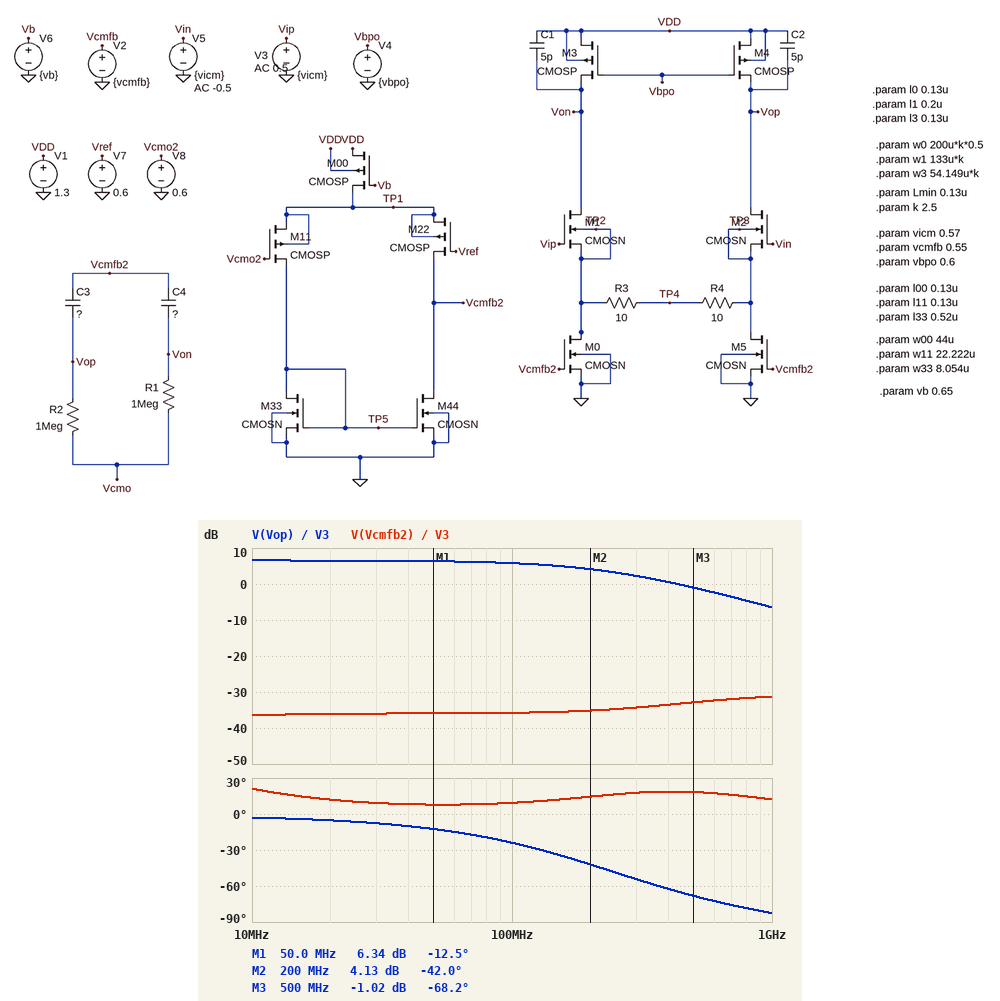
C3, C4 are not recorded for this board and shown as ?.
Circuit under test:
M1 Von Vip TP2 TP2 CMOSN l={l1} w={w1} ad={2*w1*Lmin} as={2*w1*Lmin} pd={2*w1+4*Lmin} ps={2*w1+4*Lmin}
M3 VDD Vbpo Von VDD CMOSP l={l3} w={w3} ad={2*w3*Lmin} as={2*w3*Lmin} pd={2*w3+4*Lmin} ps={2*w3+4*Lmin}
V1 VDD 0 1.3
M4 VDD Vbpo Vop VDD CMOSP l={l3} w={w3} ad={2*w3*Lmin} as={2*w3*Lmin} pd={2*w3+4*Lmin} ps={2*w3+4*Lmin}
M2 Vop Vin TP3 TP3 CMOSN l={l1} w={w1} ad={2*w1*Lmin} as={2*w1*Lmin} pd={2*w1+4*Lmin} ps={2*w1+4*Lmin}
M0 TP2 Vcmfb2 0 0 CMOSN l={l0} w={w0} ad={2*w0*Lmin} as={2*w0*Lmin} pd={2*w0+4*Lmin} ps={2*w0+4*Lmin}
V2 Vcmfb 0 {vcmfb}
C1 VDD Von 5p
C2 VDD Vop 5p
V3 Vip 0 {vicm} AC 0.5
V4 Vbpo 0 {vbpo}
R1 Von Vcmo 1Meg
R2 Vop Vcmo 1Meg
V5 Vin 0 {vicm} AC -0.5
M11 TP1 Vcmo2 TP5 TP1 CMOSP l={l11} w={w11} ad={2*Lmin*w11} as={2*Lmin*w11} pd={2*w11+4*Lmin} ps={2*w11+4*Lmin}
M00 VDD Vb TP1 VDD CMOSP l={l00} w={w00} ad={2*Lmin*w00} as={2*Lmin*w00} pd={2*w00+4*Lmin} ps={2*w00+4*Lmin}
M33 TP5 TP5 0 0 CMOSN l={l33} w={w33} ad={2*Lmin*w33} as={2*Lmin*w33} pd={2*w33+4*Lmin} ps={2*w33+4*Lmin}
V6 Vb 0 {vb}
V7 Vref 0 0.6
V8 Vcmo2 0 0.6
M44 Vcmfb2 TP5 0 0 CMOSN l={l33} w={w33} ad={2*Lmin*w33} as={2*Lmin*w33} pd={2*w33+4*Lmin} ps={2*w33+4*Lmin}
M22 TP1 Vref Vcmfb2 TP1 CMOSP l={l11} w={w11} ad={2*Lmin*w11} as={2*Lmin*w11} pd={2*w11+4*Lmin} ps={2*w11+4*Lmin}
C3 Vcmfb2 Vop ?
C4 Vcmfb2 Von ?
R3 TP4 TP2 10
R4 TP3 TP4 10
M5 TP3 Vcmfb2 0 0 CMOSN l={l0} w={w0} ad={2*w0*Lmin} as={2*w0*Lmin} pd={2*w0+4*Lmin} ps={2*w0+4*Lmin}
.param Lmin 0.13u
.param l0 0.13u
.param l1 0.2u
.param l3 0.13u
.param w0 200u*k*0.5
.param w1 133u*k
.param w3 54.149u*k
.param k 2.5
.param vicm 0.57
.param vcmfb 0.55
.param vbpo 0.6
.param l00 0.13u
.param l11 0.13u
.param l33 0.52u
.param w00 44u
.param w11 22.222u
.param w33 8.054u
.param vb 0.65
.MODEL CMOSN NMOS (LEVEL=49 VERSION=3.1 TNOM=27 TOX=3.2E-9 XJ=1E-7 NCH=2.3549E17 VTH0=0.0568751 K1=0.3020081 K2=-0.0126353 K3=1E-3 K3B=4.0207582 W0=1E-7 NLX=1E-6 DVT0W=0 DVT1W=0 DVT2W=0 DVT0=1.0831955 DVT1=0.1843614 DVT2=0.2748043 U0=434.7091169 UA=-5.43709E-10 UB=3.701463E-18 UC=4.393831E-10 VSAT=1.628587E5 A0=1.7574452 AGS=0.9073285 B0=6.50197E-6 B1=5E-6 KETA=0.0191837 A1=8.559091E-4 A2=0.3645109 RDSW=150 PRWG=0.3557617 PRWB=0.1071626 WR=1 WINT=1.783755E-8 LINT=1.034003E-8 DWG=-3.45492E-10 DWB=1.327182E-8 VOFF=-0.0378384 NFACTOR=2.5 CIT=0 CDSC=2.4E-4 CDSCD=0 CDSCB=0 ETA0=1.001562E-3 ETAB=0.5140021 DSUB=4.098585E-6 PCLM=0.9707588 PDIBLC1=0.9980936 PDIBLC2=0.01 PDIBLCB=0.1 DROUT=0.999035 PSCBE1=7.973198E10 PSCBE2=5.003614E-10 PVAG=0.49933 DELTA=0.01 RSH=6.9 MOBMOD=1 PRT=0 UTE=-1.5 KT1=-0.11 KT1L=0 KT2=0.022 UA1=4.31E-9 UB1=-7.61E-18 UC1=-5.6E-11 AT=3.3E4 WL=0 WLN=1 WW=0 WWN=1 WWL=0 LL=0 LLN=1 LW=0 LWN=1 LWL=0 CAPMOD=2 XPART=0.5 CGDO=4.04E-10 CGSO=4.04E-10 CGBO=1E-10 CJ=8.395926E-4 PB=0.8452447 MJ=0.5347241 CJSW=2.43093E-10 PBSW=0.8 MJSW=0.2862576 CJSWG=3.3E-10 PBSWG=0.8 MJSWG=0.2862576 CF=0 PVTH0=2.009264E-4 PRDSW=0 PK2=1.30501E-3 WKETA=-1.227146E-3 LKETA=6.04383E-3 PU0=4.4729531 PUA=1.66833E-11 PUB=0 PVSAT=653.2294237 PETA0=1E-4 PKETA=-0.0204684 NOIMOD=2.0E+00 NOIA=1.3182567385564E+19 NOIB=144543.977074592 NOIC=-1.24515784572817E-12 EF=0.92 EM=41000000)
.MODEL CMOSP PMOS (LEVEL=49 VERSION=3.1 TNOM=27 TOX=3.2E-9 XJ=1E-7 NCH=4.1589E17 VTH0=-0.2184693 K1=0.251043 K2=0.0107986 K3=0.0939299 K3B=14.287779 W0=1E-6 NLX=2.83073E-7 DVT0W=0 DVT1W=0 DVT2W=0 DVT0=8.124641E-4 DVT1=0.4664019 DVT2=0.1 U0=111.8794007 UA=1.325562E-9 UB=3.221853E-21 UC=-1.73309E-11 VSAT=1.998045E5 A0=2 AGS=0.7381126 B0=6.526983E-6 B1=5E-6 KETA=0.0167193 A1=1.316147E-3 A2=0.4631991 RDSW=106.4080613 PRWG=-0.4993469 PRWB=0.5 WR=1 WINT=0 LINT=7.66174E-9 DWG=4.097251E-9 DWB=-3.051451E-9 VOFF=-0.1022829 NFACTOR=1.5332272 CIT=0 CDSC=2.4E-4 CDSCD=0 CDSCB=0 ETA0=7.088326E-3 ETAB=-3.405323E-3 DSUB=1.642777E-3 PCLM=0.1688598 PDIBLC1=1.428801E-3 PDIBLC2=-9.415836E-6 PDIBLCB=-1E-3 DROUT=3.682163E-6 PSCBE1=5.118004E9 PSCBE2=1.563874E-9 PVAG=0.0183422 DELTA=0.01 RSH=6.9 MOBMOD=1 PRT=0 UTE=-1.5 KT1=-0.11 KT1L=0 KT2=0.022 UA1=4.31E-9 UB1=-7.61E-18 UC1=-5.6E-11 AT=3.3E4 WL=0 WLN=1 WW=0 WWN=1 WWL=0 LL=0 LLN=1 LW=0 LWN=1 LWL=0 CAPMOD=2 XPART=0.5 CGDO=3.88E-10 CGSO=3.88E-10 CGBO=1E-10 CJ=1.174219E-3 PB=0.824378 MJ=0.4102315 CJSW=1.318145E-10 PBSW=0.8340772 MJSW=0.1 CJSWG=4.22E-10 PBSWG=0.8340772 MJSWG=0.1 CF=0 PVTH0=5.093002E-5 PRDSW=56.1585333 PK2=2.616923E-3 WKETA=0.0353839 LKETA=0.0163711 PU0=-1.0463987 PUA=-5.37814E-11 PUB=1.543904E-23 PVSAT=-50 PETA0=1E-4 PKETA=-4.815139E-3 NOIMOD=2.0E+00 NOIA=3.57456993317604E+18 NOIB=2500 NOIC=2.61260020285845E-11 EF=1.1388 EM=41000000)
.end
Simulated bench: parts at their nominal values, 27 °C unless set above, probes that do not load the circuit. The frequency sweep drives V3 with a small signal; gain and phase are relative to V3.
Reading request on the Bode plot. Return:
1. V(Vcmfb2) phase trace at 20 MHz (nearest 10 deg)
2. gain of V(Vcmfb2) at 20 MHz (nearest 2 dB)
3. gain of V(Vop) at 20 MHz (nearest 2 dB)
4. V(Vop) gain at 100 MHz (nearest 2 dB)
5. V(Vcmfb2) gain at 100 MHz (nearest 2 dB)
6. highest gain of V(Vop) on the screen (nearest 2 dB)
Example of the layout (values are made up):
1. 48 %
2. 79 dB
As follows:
1. 10 deg
2. -36 dB
3. 6 dB
4. 6 dB
5. -36 dB
6. 6 dB
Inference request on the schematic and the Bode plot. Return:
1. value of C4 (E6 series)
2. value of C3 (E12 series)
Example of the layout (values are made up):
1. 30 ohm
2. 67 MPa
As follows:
1. 330 fF
2. 390 fF
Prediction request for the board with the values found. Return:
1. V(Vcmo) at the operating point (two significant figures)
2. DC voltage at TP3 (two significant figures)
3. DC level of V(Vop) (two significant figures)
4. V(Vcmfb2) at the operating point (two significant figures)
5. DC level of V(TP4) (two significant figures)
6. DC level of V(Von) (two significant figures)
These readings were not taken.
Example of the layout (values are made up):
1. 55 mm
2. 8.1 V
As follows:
1. 1.1 V
2. 130 mV
3. 1.1 V
4. 550 mV
5. 130 mV
6. 1.1 V
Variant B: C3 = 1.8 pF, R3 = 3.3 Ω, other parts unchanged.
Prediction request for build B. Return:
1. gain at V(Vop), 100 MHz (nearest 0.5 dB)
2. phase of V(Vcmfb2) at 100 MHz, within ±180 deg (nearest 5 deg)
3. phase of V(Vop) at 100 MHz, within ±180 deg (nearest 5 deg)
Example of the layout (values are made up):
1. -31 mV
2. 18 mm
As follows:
1. 1.5 dB
2. -10 deg
3. -20 deg
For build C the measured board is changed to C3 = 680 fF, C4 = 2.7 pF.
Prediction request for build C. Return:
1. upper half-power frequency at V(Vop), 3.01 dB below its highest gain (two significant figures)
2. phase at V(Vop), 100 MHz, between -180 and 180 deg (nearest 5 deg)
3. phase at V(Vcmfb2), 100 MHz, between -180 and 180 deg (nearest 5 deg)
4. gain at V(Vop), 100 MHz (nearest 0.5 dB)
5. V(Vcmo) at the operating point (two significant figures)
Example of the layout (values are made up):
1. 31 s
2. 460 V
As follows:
1. 200 MHz
2. -30 deg
3. 170 deg
4. 9.5 dB
5. 1.1 V
